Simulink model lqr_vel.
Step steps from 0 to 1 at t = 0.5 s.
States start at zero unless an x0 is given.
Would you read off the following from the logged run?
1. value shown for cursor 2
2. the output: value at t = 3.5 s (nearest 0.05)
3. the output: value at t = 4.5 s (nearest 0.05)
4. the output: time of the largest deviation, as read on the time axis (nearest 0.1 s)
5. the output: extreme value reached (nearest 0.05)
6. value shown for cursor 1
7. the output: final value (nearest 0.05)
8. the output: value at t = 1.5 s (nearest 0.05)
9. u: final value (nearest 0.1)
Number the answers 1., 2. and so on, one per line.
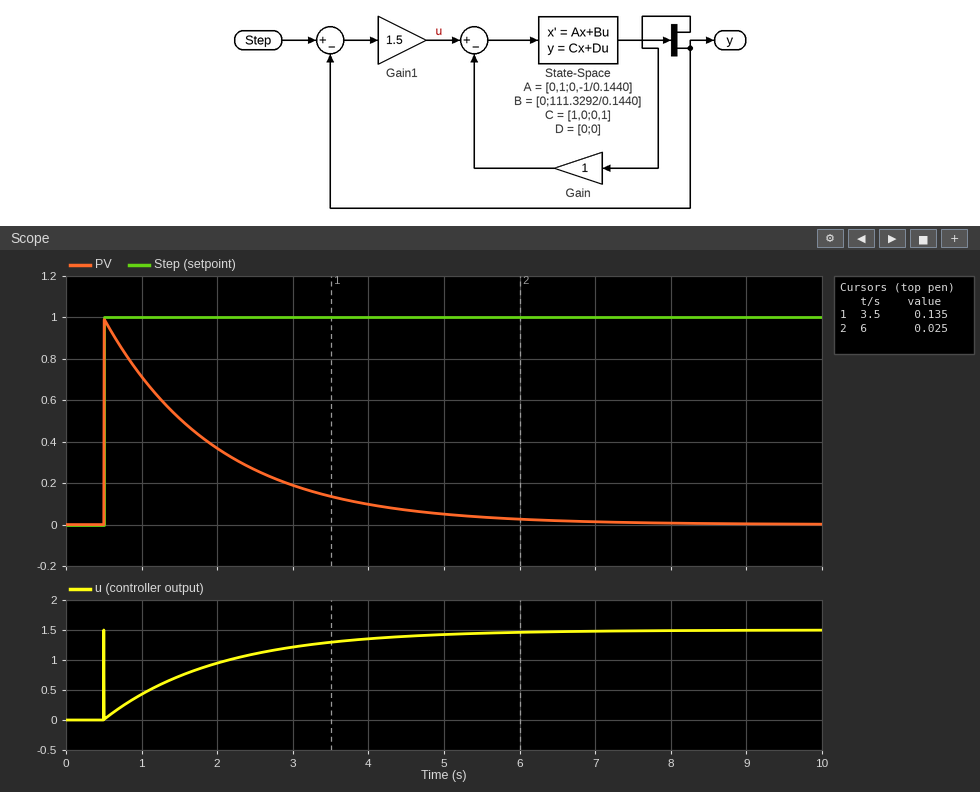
1. 0.025
2. 0.15
3. 0.05
4. 0.5 s
5. 1.00
6. 0.135
7. 0.00
8. 0.50
9. 1.5
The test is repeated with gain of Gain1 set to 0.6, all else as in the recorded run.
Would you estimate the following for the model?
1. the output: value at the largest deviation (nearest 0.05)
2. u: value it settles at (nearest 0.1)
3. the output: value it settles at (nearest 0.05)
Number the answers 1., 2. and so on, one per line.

1. 0.95
2. 0.6
3. 0.00
